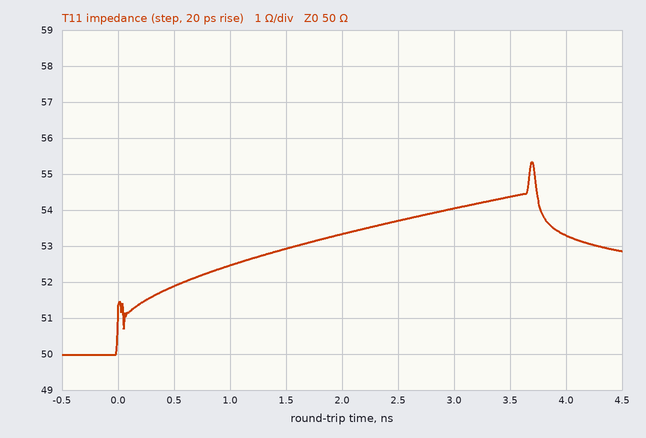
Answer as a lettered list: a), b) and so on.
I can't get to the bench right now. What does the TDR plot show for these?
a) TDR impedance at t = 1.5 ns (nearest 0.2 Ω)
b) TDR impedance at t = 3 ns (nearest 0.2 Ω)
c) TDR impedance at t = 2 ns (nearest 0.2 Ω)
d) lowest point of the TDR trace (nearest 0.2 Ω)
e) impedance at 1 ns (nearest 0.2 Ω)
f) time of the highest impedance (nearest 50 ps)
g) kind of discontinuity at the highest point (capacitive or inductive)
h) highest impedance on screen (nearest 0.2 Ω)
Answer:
a) 53.0 Ω
b) 54.0 Ω
c) 53.4 Ω
d) 50.0 Ω
e) 52.4 Ω
f) 3.70 ns
g) inductive
h) 55.4 Ω
